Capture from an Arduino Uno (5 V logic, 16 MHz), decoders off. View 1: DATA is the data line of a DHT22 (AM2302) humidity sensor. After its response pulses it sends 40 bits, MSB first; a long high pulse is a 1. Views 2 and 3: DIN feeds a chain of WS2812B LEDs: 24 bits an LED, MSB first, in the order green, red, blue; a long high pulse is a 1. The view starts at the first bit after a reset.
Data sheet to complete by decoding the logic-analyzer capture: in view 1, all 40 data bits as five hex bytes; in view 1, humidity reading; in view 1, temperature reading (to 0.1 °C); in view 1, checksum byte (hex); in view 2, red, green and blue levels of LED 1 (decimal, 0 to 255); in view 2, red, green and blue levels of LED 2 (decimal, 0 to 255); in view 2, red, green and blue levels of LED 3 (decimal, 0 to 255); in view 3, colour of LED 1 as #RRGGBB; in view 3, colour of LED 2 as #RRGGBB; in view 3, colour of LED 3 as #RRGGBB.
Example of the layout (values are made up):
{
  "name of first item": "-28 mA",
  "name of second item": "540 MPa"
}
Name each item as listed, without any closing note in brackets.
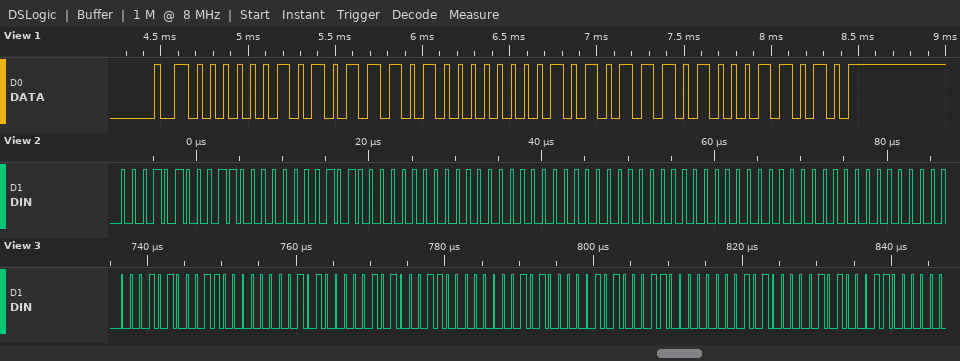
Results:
{
  "in view 1, all 40 data bits as five hex bytes": "02 BA 01 5D 1A",
  "in view 1, humidity reading": "69.8 %",
  "in view 1, temperature reading": "34.9 °C",
  "in view 1, checksum byte": "0x1A",
  "in view 2, red, green and blue levels of LED 1": "96, 20, 20",
  "in view 2, red, green and blue levels of LED 2": "0, 0, 0",
  "in view 2, red, green and blue levels of LED 3": "0, 0, 0",
  "in view 3, colour of LED 1 as #RRGGBB": "#601414",
  "in view 3, colour of LED 2 as #RRGGBB": "#601414",
  "in view 3, colour of LED 3 as #RRGGBB": "#601414"
}
